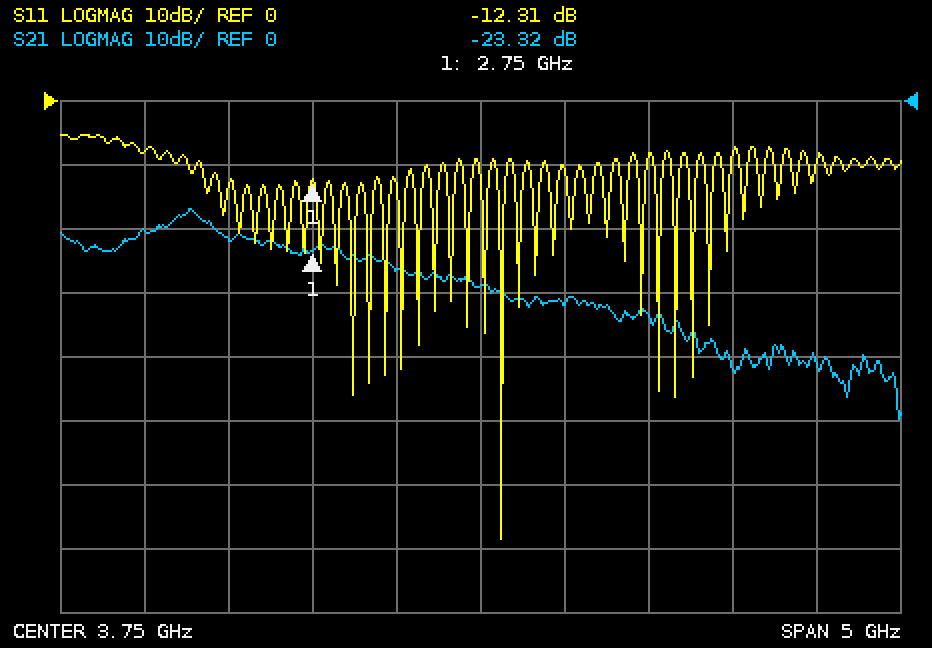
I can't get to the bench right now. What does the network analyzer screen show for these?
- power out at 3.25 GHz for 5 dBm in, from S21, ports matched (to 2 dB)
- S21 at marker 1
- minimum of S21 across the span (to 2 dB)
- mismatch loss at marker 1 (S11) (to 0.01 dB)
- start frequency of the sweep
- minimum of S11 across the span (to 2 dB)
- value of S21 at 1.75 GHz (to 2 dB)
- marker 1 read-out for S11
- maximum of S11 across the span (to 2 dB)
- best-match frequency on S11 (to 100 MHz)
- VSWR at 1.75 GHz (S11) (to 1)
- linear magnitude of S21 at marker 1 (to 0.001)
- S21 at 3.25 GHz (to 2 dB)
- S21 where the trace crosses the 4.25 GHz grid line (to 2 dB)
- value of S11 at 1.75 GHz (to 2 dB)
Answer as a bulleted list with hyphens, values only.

- -22 dBm
- -23.32 dB
- -50 dB
- 0.26 dB
- 1.25 GHz
- -68 dB
- -20 dB
- -12.31 dB
- -6 dB
- 3.9 GHz
- 2
- 0.068
- -26 dB
- -32 dB
- -8 dB
